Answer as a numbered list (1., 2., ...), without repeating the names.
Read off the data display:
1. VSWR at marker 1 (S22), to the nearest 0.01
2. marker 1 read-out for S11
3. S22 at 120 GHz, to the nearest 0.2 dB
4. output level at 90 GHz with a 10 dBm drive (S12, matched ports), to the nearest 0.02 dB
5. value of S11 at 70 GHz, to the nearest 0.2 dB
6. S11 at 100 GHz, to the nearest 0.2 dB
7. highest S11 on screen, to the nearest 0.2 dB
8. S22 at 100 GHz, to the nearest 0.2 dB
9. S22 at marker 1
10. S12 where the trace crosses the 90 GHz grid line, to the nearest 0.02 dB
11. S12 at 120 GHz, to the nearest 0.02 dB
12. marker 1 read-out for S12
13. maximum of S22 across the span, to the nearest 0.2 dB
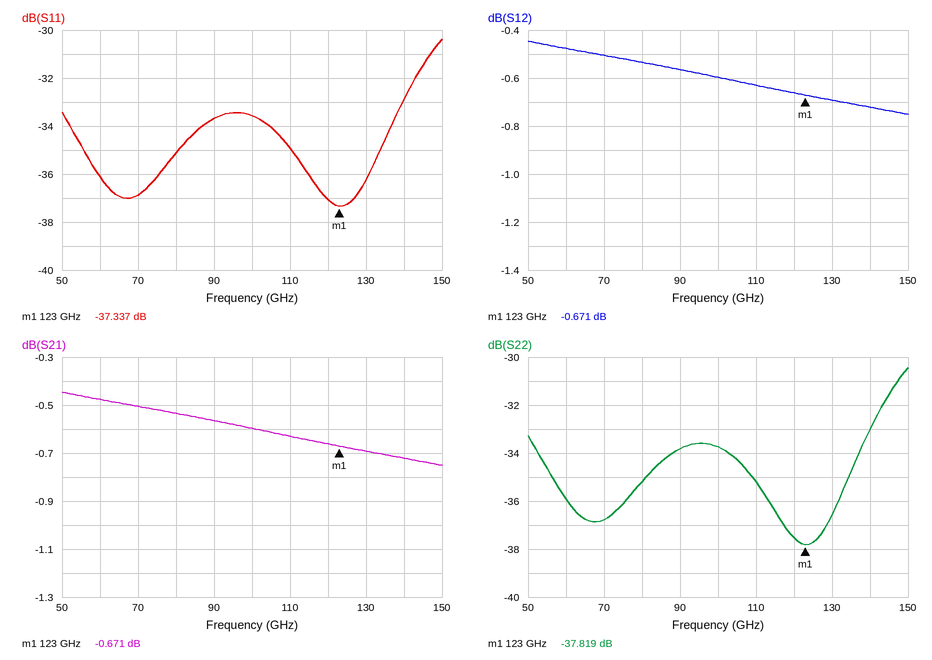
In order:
1. 1.03
2. -37.337 dB
3. -37.6 dB
4. 9.44 dBm
5. -36.8 dB
6. -33.6 dB
7. -30.4 dB
8. -33.8 dB
9. -37.819 dB
10. -0.56 dB
11. -0.66 dB
12. -0.671 dB
13. -30.4 dB
